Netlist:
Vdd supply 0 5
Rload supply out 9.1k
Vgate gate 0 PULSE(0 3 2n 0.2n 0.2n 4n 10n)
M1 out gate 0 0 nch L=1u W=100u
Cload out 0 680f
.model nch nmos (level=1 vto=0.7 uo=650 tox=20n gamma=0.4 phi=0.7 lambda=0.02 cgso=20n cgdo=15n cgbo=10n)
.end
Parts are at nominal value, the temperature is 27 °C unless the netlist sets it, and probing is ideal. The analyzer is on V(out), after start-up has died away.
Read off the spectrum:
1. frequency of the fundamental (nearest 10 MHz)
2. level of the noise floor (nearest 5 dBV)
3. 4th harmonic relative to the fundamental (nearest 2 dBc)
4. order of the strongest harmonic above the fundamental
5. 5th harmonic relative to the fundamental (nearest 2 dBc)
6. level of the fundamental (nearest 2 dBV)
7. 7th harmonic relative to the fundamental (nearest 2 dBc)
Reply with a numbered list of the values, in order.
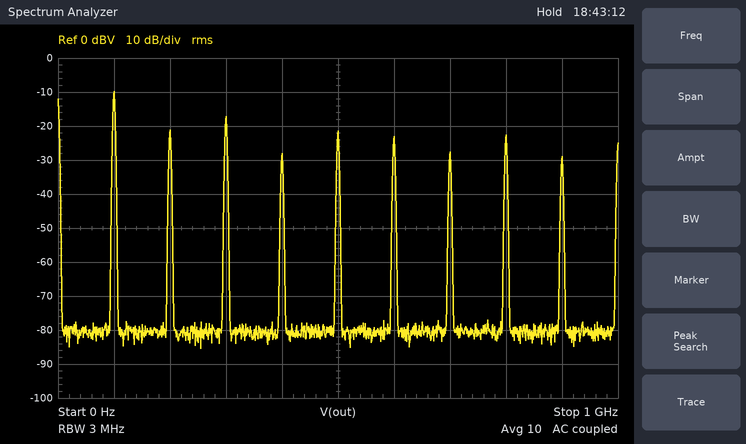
1. 100 MHz
2. -80 dBV
3. -18 dBc
4. 3
5. -12 dBc
6. -10 dBV
7. -18 dBc
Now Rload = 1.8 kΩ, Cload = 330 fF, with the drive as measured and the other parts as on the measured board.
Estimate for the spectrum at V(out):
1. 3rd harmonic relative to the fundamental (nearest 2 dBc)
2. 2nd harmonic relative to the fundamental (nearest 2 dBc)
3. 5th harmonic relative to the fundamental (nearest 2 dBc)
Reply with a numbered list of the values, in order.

1. -10 dBc
2. -12 dBc
3. -16 dBc
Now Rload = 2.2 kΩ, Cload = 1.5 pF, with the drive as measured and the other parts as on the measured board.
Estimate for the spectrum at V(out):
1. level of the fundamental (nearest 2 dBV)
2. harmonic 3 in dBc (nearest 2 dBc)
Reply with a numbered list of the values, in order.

1. -2 dBV
2. -10 dBc
